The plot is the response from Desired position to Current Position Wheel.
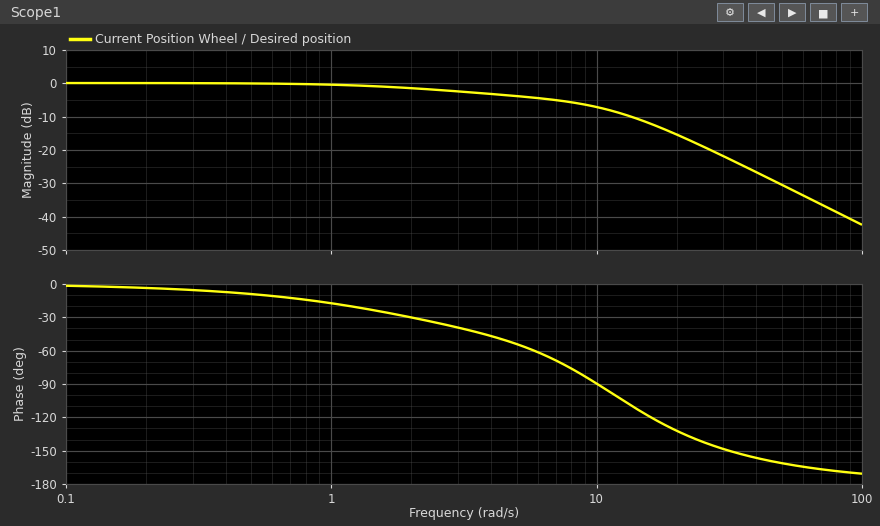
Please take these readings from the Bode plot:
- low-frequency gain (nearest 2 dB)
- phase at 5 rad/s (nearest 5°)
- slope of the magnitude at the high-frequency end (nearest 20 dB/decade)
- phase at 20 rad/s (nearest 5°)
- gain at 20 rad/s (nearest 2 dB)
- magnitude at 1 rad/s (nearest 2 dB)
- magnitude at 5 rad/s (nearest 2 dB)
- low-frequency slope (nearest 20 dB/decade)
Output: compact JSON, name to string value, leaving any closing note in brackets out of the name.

{"low-frequency gain": "0 dB", "phase at 5 rad/s": "-55°", "slope of the magnitude at the high-frequency end": "-40 dB/decade", "phase at 20 rad/s": "-130°", "gain at 20 rad/s": "-16 dB", "magnitude at 1 rad/s": "0 dB", "magnitude at 5 rad/s": "-4 dB", "low-frequency slope": "0 dB/decade"}
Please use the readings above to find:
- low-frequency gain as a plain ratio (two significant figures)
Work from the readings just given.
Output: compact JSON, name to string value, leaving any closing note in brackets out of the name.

{"low-frequency gain as a plain ratio": "1.0"}
